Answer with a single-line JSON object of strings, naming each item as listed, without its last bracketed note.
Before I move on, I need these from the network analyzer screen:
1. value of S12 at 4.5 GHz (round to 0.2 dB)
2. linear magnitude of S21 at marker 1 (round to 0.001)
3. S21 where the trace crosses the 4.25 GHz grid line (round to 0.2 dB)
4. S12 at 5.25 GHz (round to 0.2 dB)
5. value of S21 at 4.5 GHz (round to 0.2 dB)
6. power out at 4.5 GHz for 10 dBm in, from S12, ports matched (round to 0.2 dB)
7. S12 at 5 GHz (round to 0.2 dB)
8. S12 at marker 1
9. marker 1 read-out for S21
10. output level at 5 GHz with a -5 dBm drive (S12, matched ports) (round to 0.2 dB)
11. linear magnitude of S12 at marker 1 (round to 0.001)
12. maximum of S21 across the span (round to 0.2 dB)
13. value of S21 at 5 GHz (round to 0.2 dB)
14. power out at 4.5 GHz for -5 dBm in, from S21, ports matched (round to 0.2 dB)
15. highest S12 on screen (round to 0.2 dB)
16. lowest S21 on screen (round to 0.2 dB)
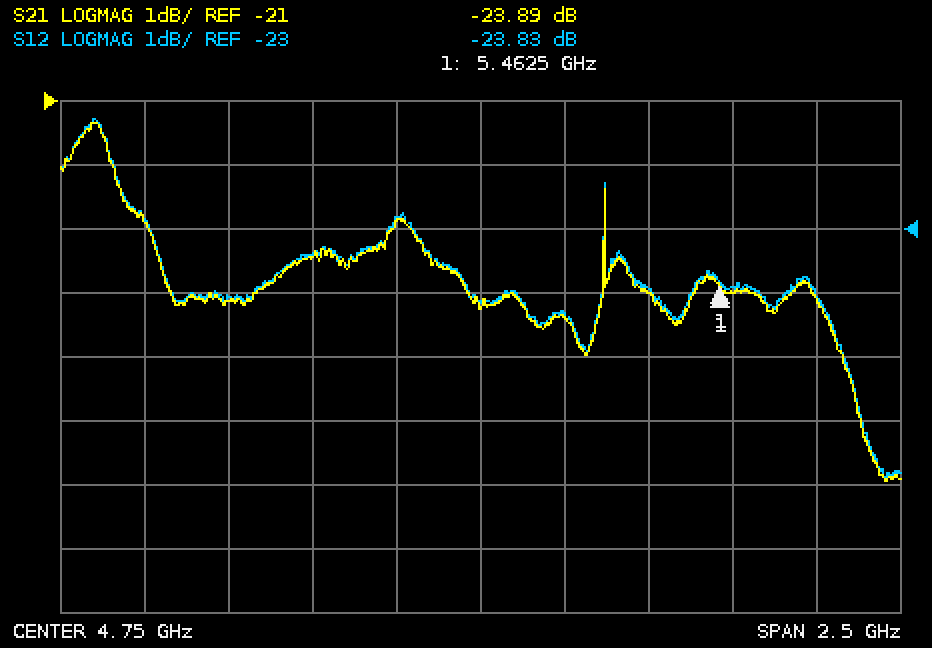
{"value of S12 at 4.5 GHz": "-22.8 dB", "linear magnitude of S21 at marker 1": "0.064", "S21 where the trace crosses the 4.25 GHz grid line": "-23.4 dB", "S12 at 5.25 GHz": "-24.0 dB", "value of S21 at 4.5 GHz": "-22.8 dB", "power out at 4.5 GHz for 10 dBm in, from S12, ports matched": "-12.8 dBm", "S12 at 5 GHz": "-24.4 dB", "S12 at marker 1": "-23.83 dB", "marker 1 read-out for S21": "-23.89 dB", "output level at 5 GHz with a -5 dBm drive (S12, matched ports)": "-29.4 dBm", "linear magnitude of S12 at marker 1": "0.064", "maximum of S21 across the span": "-21.4 dB", "value of S21 at 5 GHz": "-24.4 dB", "power out at 4.5 GHz for -5 dBm in, from S21, ports matched": "-27.8 dBm", "highest S12 on screen": "-21.2 dB", "lowest S21 on screen": "-27.0 dB"}
